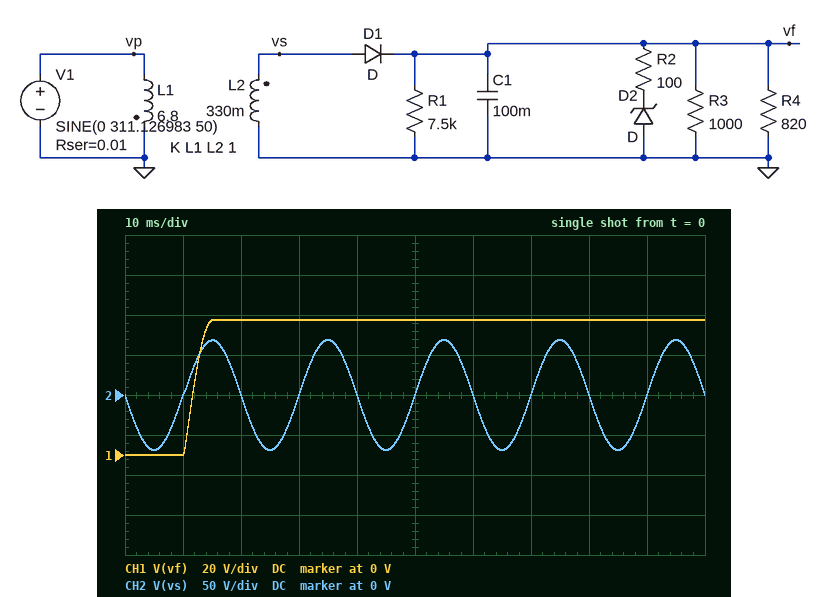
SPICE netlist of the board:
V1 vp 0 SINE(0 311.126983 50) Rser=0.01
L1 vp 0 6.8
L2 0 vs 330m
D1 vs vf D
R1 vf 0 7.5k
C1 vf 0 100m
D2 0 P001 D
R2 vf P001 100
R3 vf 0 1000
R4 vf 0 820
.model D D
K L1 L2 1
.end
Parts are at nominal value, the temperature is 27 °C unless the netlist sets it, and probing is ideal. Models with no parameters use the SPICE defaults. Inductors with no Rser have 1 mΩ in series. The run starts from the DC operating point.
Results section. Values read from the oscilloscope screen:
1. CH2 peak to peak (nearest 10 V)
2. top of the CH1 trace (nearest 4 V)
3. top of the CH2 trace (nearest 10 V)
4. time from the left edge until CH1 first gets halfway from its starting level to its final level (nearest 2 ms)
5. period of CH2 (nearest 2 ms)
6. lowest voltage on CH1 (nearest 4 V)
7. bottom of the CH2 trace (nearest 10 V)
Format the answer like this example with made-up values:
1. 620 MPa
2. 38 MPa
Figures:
1. 140 V
2. 68 V
3. 70 V
4. 12 ms
5. 20 ms
6. 0 V
7. -70 V
